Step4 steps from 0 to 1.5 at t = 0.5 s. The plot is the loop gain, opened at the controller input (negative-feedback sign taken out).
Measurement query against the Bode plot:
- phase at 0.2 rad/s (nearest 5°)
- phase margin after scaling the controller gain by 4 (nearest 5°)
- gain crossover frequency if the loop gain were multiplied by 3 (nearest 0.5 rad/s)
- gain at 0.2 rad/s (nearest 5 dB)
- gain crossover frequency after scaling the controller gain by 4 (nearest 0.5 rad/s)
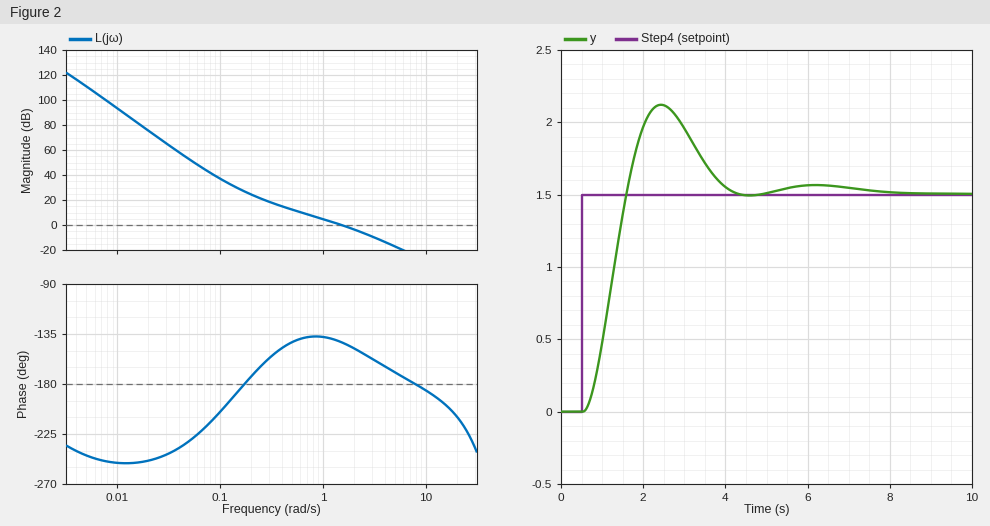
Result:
-175°
20°
3.0 rad/s
25 dB
3.5 rad/s
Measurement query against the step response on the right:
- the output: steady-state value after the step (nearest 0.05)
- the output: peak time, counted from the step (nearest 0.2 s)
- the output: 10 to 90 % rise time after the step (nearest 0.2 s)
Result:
1.50
2.0 s
0.8 s
